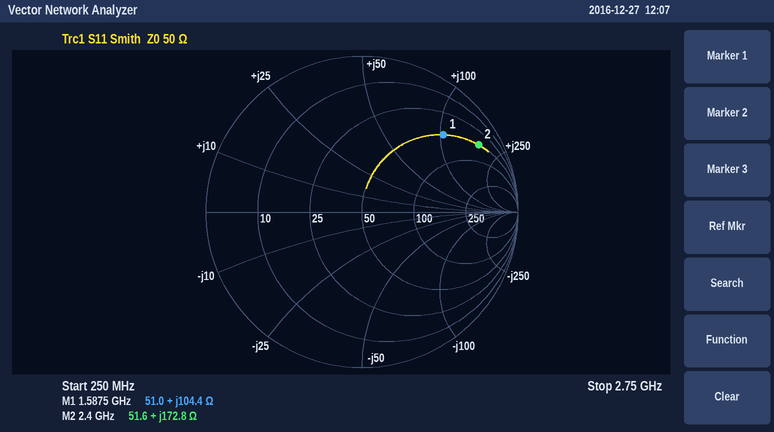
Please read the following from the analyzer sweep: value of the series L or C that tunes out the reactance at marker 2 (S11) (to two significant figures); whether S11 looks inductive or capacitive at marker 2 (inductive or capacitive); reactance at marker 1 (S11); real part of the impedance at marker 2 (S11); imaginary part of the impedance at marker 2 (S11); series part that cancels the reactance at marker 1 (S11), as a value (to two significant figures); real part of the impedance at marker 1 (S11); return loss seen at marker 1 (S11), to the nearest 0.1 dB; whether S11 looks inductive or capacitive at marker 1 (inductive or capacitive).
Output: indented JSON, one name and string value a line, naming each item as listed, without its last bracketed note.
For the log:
{
  "value of the series L or C that tunes out the reactance at marker 2 (S11)": "380 fF",
  "whether S11 looks inductive or capacitive at marker 2": "inductive",
  "reactance at marker 1": "+104.4 Ω",
  "real part of the impedance at marker 2": "51.6 Ω",
  "imaginary part of the impedance at marker 2": "+172.8 Ω",
  "series part that cancels the reactance at marker 1 (S11), as a value": "960 fF",
  "real part of the impedance at marker 1": "51.0 Ω",
  "return loss seen at marker 1 (S11), to the nearest 0.1 dB": "2.9 dB",
  "whether S11 looks inductive or capacitive at marker 1": "inductive"
}
